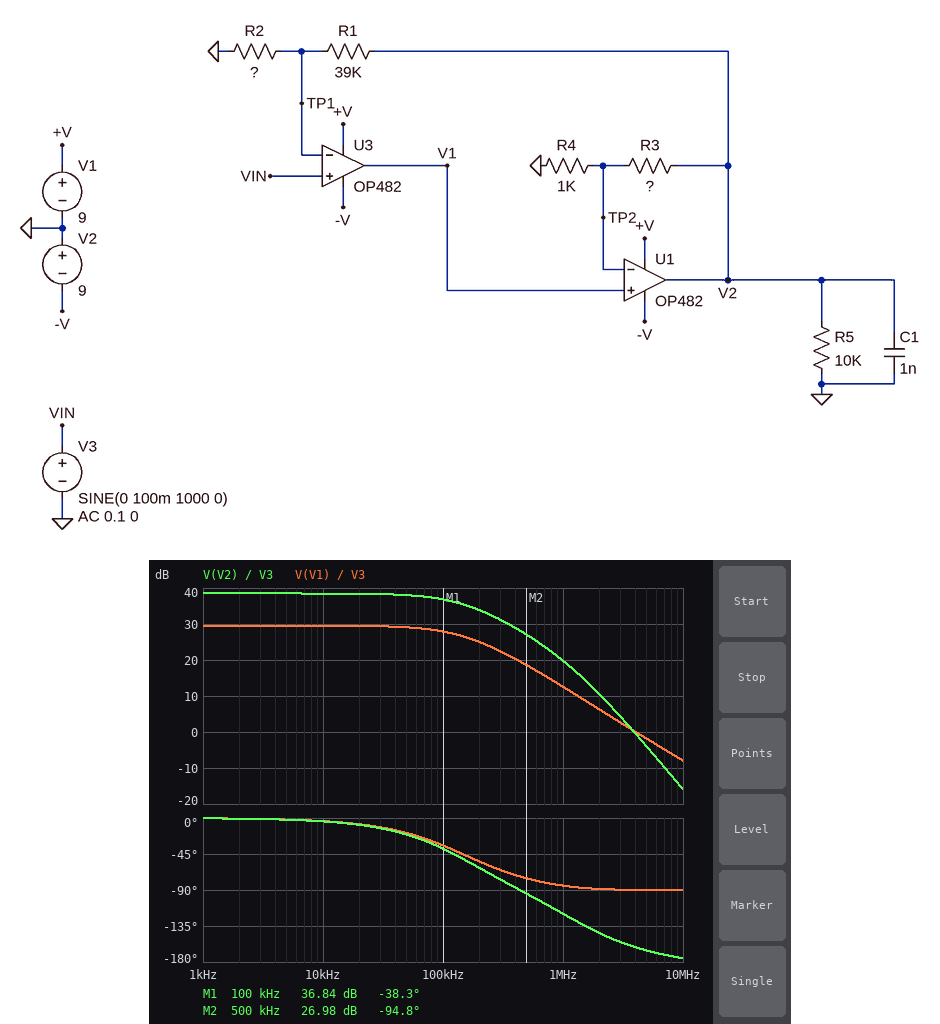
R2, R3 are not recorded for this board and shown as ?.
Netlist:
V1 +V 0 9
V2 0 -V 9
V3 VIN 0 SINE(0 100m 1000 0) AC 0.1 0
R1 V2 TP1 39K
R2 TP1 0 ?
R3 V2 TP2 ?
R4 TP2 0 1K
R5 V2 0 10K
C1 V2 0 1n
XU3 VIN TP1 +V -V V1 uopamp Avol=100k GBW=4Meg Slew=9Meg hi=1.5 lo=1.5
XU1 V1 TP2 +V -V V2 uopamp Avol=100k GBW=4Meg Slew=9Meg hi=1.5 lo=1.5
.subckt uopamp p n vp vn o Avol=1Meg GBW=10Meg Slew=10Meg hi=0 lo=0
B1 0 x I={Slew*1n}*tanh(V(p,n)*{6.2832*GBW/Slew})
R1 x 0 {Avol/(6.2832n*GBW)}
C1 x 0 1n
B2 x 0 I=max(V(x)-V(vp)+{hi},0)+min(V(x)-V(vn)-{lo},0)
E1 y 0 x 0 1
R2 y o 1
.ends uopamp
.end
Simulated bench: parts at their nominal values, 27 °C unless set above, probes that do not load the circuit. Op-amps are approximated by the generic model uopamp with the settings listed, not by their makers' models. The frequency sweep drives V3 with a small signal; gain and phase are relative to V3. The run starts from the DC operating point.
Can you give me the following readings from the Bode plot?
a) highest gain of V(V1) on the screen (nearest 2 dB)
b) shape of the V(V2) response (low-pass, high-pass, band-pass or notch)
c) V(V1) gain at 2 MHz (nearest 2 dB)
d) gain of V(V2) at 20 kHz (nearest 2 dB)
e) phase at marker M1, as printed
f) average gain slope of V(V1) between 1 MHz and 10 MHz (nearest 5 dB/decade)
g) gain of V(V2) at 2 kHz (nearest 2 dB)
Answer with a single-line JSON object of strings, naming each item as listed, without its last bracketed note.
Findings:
{"highest gain of V(V1) on the screen": "30 dB", "shape of the V(V2) response": "low-pass", "V(V1) gain at 2 MHz": "6 dB", "gain of V(V2) at 20 kHz": "38 dB", "phase at marker M1, as printed": "-38.3 deg", "average gain slope of V(V1) between 1 MHz and 10 MHz": "-20 dB/decade", "gain of V(V2) at 2 kHz": "38 dB"}
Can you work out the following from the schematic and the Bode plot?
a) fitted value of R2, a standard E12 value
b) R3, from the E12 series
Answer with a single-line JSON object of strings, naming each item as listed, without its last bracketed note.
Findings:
{"fitted value of R2, a standard E12 value": "470 Ω", "R3, from the E12 series": "1.8 kΩ"}
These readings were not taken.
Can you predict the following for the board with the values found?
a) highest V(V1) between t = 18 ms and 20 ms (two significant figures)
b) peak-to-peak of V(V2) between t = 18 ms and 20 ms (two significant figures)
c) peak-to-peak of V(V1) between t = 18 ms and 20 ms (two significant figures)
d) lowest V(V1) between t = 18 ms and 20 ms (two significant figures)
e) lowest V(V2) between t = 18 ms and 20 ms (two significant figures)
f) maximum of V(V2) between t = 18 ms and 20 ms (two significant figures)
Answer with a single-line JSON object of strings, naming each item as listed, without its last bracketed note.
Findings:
{"highest V(V1) between t = 18 ms and 20 ms": "7.5 V", "peak-to-peak of V(V2) between t = 18 ms and 20 ms": "15 V", "peak-to-peak of V(V1) between t = 18 ms and 20 ms": "15 V", "lowest V(V1) between t = 18 ms and 20 ms": "-7.5 V", "lowest V(V2) between t = 18 ms and 20 ms": "-7.5 V", "maximum of V(V2) between t = 18 ms and 20 ms": "7.5 V"}
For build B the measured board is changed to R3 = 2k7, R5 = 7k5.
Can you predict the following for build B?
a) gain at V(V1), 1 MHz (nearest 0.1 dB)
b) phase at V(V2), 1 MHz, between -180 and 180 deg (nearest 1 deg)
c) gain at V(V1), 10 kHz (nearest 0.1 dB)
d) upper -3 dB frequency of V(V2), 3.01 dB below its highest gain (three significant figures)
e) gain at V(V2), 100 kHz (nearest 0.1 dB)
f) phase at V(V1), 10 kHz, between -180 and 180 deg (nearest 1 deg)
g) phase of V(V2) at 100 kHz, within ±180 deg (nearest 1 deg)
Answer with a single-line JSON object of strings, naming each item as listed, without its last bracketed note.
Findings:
{"gain at V(V1), 1 MHz": "12.8 dB", "phase at V(V2), 1 MHz, between -180 and 180 deg": "-127 deg", "gain at V(V1), 10 kHz": "27.1 dB", "upper -3 dB frequency of V(V2), 3.01 dB below its highest gain": "209 kHz", "gain at V(V2), 100 kHz": "37.6 dB", "phase at V(V1), 10 kHz, between -180 and 180 deg": "-3 deg", "phase of V(V2) at 100 kHz, within ±180 deg": "-31 deg"}
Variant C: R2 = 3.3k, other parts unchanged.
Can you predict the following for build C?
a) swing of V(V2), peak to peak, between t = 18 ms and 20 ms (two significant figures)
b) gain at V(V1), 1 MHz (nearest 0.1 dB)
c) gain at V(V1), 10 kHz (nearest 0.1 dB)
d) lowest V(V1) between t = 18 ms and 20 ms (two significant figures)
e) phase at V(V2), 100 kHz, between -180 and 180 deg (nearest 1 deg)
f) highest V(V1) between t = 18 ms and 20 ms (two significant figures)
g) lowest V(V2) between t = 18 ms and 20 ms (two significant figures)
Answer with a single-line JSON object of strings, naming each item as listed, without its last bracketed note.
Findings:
{"swing of V(V2), peak to peak, between t = 18 ms and 20 ms": "2.6 V", "gain at V(V1), 1 MHz": "13.7 dB", "gain at V(V1), 10 kHz": "13.2 dB", "lowest V(V1) between t = 18 ms and 20 ms": "-460 mV", "phase at V(V2), 100 kHz, between -180 and 180 deg": "-7 deg", "highest V(V1) between t = 18 ms and 20 ms": "460 mV", "lowest V(V2) between t = 18 ms and 20 ms": "-1.3 V"}
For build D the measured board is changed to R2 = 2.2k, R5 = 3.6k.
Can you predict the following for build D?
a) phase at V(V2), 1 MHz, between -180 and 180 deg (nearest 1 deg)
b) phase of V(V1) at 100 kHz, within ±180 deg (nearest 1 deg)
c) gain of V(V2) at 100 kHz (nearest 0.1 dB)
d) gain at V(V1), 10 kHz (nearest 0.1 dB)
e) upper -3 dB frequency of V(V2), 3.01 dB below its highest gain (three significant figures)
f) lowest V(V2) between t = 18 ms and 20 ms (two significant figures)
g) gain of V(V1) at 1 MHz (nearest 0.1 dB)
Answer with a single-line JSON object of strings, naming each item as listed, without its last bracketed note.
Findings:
{"phase at V(V2), 1 MHz, between -180 and 180 deg": "-96 deg", "phase of V(V1) at 100 kHz, within ±180 deg": "-6 deg", "gain of V(V2) at 100 kHz": "25.4 dB", "gain at V(V1), 10 kHz": "16.5 dB", "upper -3 dB frequency of V(V2), 3.01 dB below its highest gain": "842 kHz", "lowest V(V2) between t = 18 ms and 20 ms": "-1.9 V", "gain of V(V1) at 1 MHz": "13.7 dB"}
